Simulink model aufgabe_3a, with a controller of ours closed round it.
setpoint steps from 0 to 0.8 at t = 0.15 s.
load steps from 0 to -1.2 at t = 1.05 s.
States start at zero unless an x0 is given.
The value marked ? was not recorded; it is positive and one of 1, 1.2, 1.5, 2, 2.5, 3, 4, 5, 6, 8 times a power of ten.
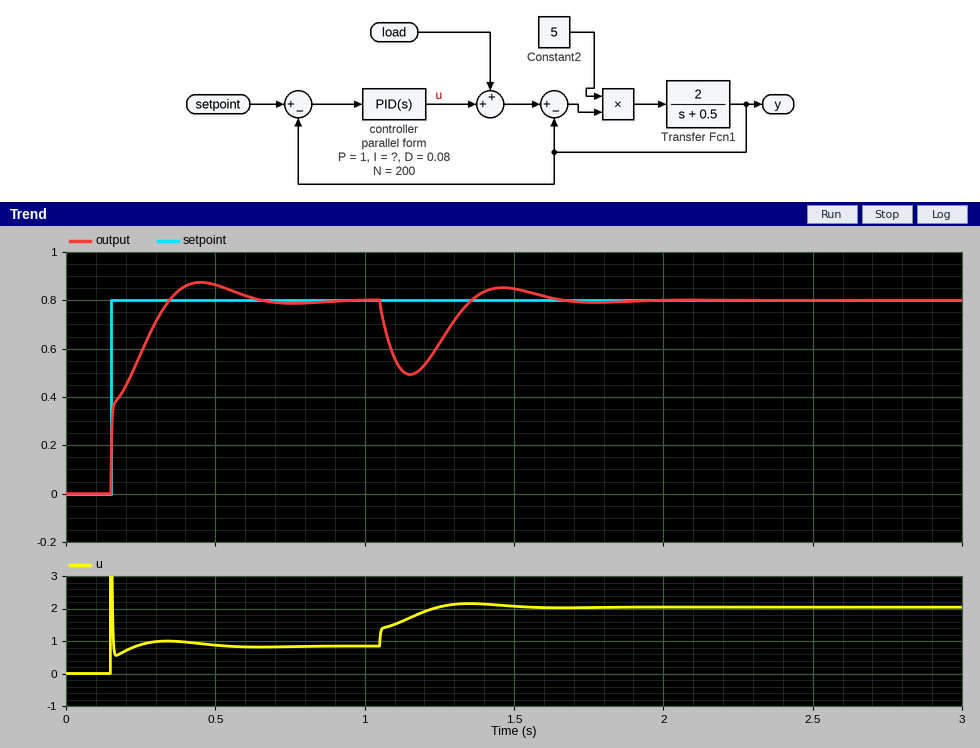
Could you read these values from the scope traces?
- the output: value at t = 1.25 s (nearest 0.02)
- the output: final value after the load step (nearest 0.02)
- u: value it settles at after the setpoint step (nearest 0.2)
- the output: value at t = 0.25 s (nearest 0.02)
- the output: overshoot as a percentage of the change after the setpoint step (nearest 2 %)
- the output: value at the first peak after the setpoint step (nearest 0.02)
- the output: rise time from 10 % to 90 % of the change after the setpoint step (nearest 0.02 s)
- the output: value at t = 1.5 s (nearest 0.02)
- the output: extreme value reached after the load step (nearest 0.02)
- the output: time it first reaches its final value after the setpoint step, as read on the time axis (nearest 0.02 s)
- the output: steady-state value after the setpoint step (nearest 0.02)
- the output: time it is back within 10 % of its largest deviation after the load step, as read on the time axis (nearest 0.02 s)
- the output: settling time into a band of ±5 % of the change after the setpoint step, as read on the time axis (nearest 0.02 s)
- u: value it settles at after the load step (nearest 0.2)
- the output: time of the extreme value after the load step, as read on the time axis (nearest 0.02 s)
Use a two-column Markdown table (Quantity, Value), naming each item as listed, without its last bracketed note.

| Quantity | Value |
|---|---|
| the output: value at t = 1.25 s | 0.62 |
| the output: final value after the load step | 0.80 |
| u: value it settles at after the setpoint step | 0.8 |
| the output: value at t = 0.25 s | 0.58 |
| the output: overshoot as a percentage of the change after the setpoint step | 10 % |
| the output: value at the first peak after the setpoint step | 0.88 |
| the output: rise time from 10 % to 90 % of the change after the setpoint step | 0.16 s |
| the output: value at t = 1.5 s | 0.84 |
| the output: extreme value reached after the load step | 0.50 |
| the output: time it first reaches its final value after the setpoint step, as read on the time axis | 0.34 s |
| the output: steady-state value after the setpoint step | 0.80 |
| the output: time it is back within 10 % of its largest deviation after the load step, as read on the time axis | 1.56 s |
| the output: settling time into a band of ±5 % of the change after the setpoint step, as read on the time axis | 0.56 s |
| u: value it settles at after the load step | 2.0 |
| the output: time of the extreme value after the load step, as read on the time axis | 1.16 s |
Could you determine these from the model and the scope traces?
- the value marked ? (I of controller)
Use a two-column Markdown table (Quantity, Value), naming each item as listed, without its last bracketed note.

| Quantity | Value |
|---|---|
| the value marked ? | 25 |
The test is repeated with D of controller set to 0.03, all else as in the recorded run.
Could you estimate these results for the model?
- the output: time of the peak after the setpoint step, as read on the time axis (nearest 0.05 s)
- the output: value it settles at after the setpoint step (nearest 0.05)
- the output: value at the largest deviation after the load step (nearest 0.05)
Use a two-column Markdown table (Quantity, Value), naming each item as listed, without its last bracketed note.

| Quantity | Value |
|---|---|
| the output: time of the peak after the setpoint step, as read on the time axis | 0.40 s |
| the output: value it settles at after the setpoint step | 0.80 |
| the output: value at the largest deviation after the load step | 0.45 |
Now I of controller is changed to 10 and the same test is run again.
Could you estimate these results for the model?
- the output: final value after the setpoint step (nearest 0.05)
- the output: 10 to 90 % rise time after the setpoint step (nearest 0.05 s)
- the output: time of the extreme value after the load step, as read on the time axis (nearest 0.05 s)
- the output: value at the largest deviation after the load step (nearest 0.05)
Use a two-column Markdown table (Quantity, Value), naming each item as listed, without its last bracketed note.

| Quantity | Value |
|---|---|
| the output: final value after the setpoint step | 0.80 |
| the output: 10 to 90 % rise time after the setpoint step | 0.30 s |
| the output: time of the extreme value after the load step, as read on the time axis | 1.20 s |
| the output: value at the largest deviation after the load step | 0.40 |
